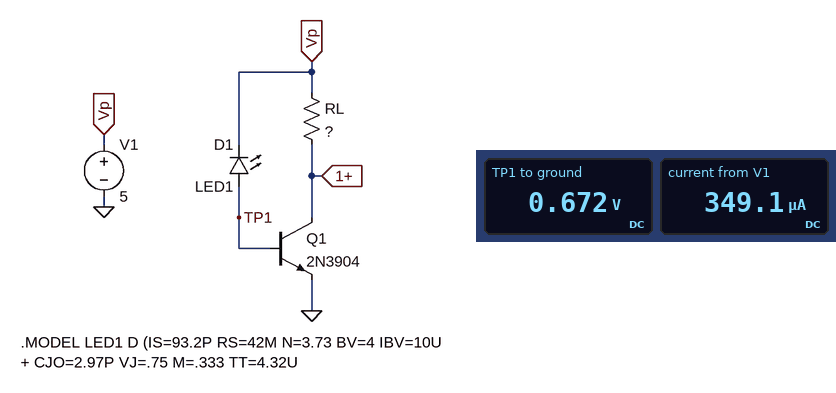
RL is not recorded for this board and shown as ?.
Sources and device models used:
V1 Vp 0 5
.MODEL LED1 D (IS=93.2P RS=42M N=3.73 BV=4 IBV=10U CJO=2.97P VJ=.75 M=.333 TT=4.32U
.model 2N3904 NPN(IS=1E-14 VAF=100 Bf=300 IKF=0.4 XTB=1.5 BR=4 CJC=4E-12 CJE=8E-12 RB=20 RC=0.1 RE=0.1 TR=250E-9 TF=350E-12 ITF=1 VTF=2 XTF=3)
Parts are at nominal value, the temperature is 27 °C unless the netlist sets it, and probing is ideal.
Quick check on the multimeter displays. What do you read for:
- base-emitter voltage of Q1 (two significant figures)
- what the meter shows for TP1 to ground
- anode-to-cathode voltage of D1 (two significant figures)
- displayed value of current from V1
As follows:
670 mV
0.672 V
-4.3 V
349.1 µA
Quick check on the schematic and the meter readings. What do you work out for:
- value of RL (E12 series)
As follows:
100 kΩ
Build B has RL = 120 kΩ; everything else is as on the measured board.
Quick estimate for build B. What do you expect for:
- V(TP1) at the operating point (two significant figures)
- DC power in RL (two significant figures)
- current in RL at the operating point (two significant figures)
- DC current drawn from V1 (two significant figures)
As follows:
670 mV
210 µW
42 µA
340 µA
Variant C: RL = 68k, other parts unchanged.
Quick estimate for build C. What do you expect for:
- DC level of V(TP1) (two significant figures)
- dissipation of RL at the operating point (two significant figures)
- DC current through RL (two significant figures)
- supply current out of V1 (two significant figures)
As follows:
670 mV
370 µW
73 µA
370 µA
